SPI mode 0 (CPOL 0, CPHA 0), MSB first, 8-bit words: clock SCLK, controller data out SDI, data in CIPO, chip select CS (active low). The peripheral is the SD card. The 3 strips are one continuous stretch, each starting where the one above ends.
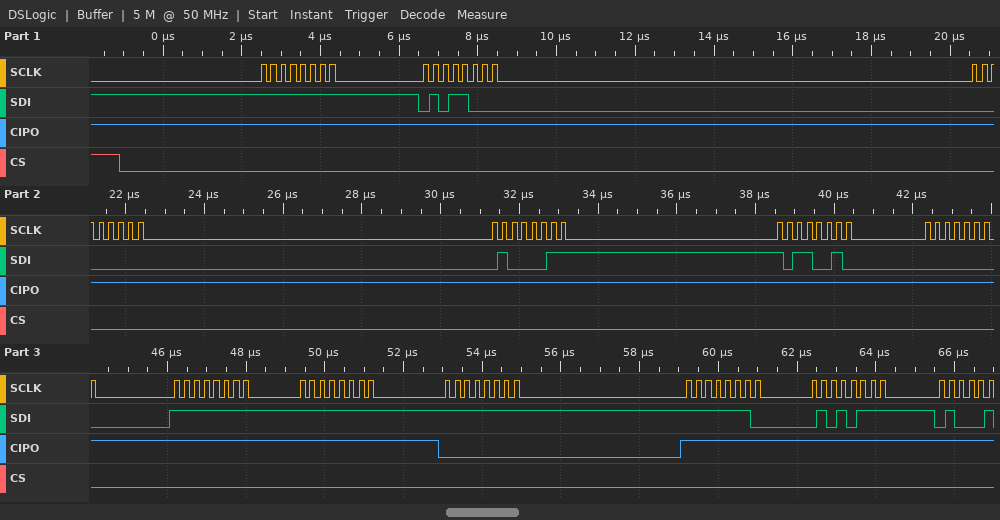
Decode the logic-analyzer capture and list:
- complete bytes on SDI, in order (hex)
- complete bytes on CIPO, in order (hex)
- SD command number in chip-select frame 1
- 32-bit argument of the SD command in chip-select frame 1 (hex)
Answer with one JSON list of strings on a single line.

["FF 58 00 43 B2 00 FF FF FF FE 57", "FF FF FF FF FF FF FF FF 00 FF FF", "CMD24", "0x0043B200"]
